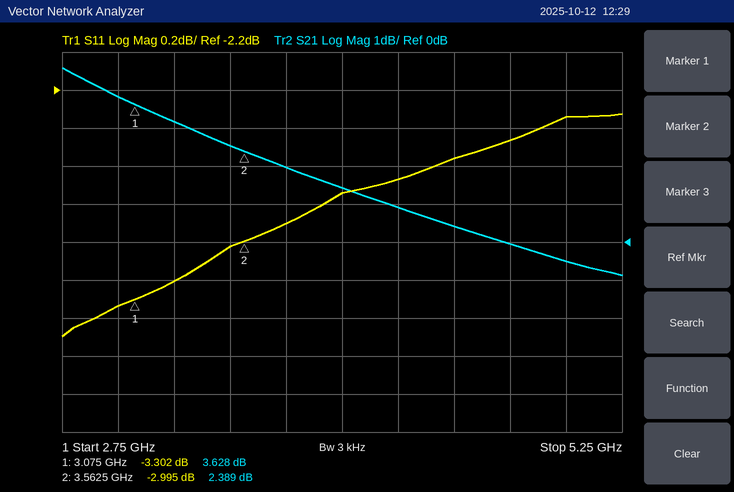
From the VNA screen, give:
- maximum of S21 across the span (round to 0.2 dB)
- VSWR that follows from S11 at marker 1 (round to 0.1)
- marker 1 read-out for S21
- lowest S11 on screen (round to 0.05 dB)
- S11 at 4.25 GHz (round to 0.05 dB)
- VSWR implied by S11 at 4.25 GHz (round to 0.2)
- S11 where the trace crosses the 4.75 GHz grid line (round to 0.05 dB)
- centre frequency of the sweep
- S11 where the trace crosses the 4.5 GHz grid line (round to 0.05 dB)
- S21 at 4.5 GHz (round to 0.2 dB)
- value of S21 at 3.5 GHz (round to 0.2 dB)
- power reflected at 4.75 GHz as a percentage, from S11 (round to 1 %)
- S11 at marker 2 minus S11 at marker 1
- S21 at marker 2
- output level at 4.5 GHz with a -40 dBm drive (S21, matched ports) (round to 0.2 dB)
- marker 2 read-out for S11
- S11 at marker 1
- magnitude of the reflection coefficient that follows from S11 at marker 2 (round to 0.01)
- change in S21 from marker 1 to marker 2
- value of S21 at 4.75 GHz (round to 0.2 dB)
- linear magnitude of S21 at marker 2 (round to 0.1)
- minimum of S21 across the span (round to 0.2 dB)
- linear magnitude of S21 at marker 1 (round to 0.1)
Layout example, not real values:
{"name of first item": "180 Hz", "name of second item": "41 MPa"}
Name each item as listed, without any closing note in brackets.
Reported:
{"maximum of S21 across the span": "4.6 dB", "VSWR that follows from S11 at marker 1": "5.3", "marker 1 read-out for S21": "3.628 dB", "lowest S11 on screen": "-3.50 dB", "S11 at 4.25 GHz": "-2.65 dB", "VSWR implied by S11 at 4.25 GHz": "6.6", "S11 where the trace crosses the 4.75 GHz grid line": "-2.45 dB", "centre frequency of the sweep": "4 GHz", "S11 where the trace crosses the 4.5 GHz grid line": "-2.55 dB", "S21 at 4.5 GHz": "0.4 dB", "value of S21 at 3.5 GHz": "2.6 dB", "power reflected at 4.75 GHz as a percentage, from S11": "57 %", "S11 at marker 2 minus S11 at marker 1": "0.307 dB", "S21 at marker 2": "2.389 dB", "output level at 4.5 GHz with a -40 dBm drive (S21, matched ports)": "-39.6 dBm", "marker 2 read-out for S11": "-2.995 dB", "S11 at marker 1": "-3.302 dB", "magnitude of the reflection coefficient that follows from S11 at marker 2": "0.71", "change in S21 from marker 1 to marker 2": "-1.239 dB", "value of S21 at 4.75 GHz": "0.0 dB", "linear magnitude of S21 at marker 2": "1.3", "minimum of S21 across the span": "-0.8 dB", "linear magnitude of S21 at marker 1": "1.5"}
